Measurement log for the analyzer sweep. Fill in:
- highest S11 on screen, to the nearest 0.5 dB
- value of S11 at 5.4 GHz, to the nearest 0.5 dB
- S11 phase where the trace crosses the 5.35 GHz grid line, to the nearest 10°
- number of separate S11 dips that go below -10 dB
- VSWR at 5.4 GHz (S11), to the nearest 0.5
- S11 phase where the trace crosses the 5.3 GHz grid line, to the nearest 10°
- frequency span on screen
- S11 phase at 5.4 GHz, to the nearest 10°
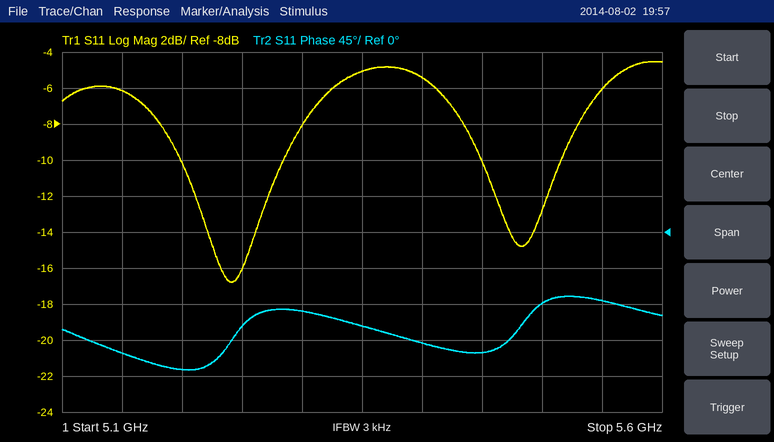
-4.5 dB
-5.5 dB
-120°
2
3.5
-100°
500 MHz
-140°
